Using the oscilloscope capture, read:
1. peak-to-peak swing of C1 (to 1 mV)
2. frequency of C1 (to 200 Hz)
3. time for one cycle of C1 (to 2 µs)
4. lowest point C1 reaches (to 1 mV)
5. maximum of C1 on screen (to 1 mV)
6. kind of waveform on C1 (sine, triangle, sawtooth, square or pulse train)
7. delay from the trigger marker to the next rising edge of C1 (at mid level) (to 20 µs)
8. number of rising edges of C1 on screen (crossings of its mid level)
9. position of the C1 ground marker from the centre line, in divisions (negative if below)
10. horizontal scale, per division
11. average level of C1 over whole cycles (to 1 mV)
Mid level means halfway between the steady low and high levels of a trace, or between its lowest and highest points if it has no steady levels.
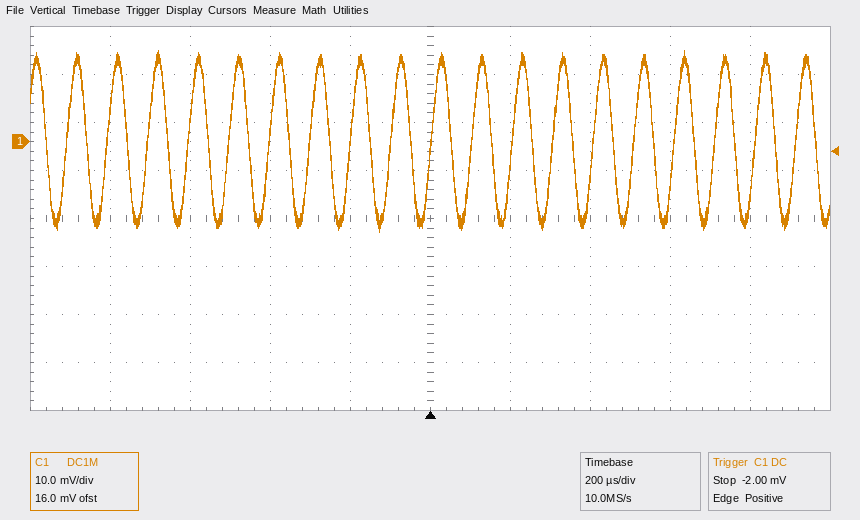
38 mV
9.8 kHz
102 µs
-19 mV
19 mV
sine
100 µs
19
+1.6 div
200 µs
0 mV
